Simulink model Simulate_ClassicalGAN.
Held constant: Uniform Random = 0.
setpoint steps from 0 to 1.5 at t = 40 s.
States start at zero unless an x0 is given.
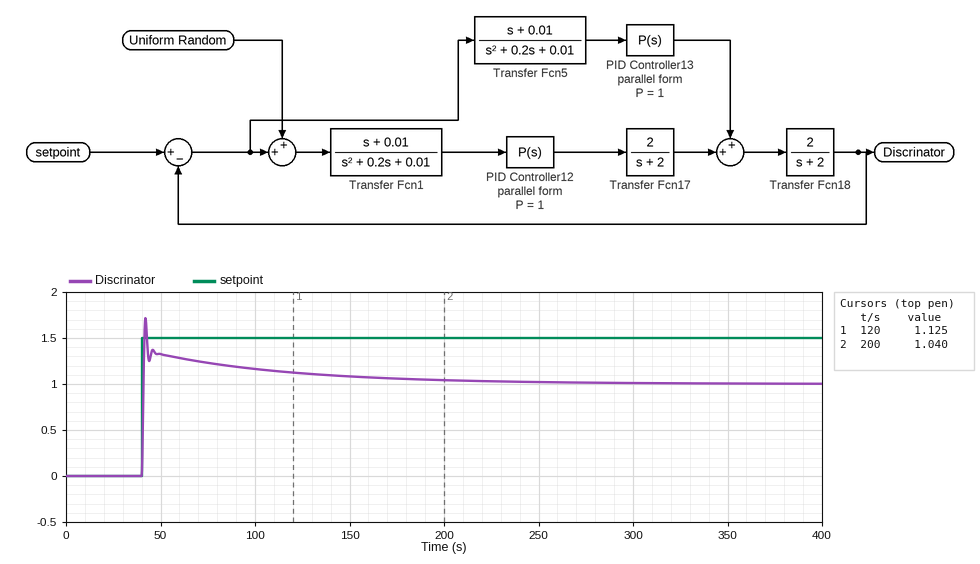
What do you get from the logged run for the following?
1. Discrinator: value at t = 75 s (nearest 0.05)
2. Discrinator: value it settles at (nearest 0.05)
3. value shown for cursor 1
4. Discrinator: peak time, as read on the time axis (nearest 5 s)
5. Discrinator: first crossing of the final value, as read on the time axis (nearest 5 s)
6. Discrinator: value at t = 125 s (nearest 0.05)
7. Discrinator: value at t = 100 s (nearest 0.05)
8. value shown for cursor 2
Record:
1.25
1.00
1.125
40 s
40 s
1.10
1.15
1.040
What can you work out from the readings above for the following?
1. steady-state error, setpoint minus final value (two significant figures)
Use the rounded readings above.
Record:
0.50
